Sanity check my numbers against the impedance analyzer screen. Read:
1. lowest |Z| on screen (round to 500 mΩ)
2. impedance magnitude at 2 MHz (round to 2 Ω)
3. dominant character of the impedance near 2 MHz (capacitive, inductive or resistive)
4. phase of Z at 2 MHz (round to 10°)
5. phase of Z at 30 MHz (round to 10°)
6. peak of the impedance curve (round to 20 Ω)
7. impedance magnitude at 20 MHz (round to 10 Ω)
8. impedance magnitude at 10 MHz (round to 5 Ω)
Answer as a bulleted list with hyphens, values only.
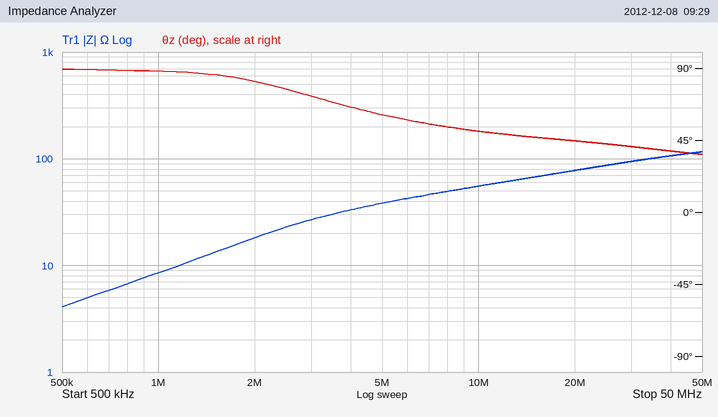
- 4.0 Ω
- 18 Ω
- inductive
- 80°
- 40°
- 120 Ω
- 80 Ω
- 55 Ω
